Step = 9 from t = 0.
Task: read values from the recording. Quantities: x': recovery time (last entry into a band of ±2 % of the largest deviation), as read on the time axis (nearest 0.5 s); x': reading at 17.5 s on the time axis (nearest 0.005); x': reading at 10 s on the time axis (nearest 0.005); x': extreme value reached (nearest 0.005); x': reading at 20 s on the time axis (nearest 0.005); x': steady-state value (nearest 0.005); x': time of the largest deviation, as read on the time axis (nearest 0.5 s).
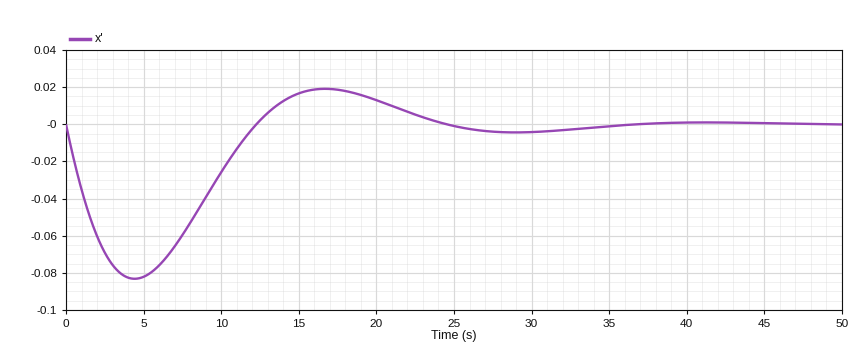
34.0 s
0.020
-0.025
-0.085
0.015
0.000
4.5 s
